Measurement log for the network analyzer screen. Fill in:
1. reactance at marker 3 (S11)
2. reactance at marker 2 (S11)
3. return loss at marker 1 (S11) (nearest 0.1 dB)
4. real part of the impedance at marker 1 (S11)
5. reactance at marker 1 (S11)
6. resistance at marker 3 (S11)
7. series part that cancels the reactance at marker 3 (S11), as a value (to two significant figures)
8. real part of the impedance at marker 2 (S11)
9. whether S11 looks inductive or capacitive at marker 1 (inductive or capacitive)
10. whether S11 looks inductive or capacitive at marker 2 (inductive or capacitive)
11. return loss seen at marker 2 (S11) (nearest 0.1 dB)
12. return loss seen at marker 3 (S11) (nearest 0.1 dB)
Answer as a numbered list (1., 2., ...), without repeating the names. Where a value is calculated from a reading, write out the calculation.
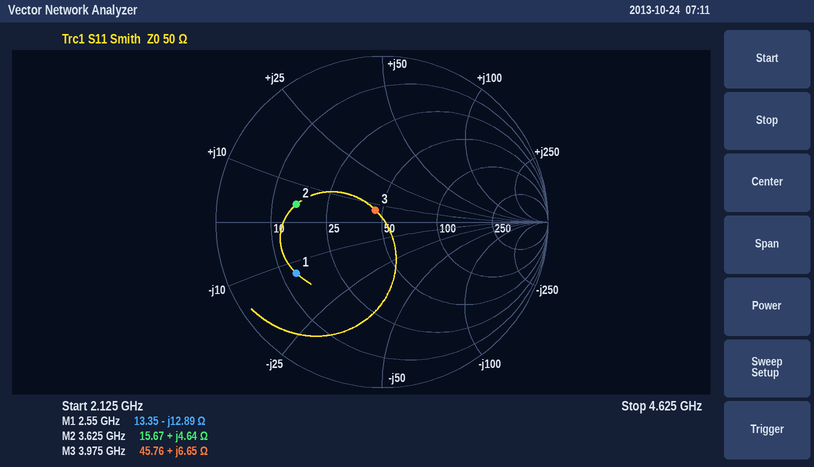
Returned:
1. +6.65 Ω
2. +4.64 Ω
3. 4.4 dB
4. 13.35 Ω
5. -12.89 Ω
6. 45.76 Ω
7. C = 1/(2π × 3.975 GHz × 6.65 Ω) ≈ 6.0 pF
8. 15.67 Ω
9. capacitive
10. inductive
11. 5.6 dB
12. 21.7 dB
